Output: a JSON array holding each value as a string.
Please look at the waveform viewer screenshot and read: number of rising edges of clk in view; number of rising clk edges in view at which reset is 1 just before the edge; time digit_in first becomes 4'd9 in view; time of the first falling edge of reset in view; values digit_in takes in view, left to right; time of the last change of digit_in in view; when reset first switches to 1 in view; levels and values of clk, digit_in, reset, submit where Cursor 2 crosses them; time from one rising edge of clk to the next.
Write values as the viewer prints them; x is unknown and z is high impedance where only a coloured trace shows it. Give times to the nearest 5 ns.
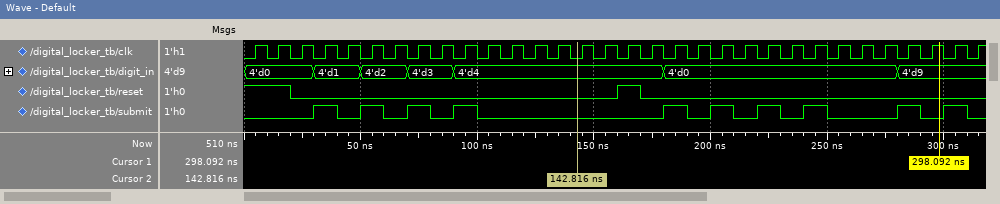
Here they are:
["32", "3", "280 ns", "20 ns", "4'd0, 4'd1, 4'd2, 4'd3, 4'd4, 4'd0, 4'd9", "280 ns", "160 ns", "clk=0, digit_in=4'd4, reset=0, submit=0", "10 ns"]
